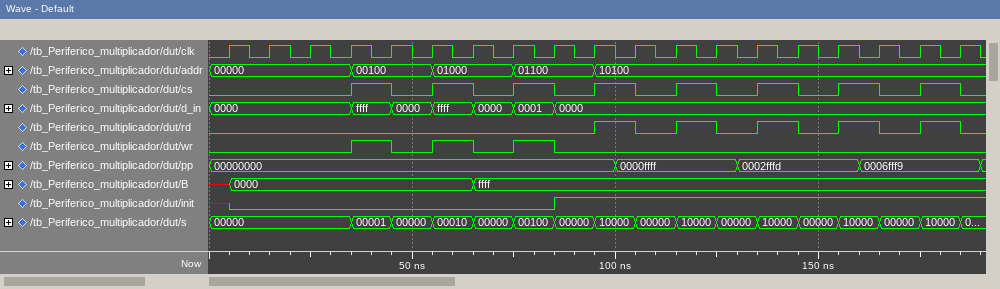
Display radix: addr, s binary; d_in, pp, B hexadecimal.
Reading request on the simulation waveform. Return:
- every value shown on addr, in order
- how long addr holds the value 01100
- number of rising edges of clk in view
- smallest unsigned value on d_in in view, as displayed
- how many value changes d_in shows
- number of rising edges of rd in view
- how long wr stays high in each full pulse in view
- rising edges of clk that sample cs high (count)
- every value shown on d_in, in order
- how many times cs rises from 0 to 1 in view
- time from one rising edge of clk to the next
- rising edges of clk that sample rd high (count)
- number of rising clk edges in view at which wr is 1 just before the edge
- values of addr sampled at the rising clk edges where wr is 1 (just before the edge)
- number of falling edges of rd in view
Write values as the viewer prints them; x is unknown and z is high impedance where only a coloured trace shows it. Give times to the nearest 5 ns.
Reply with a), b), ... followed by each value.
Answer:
a) 00000, 00100, 01000, 01100, 10100
b) 20 ns
c) 19
d) 0000
e) 6
f) 5
g) 10 ns, 10 ns, 10 ns
h) 8
i) 0000, ffff, 0000, ffff, 0000, 0001, 0000
j) 8
k) 10 ns
l) 5
m) 3
n) 00100, 01000, 01100
o) 5
